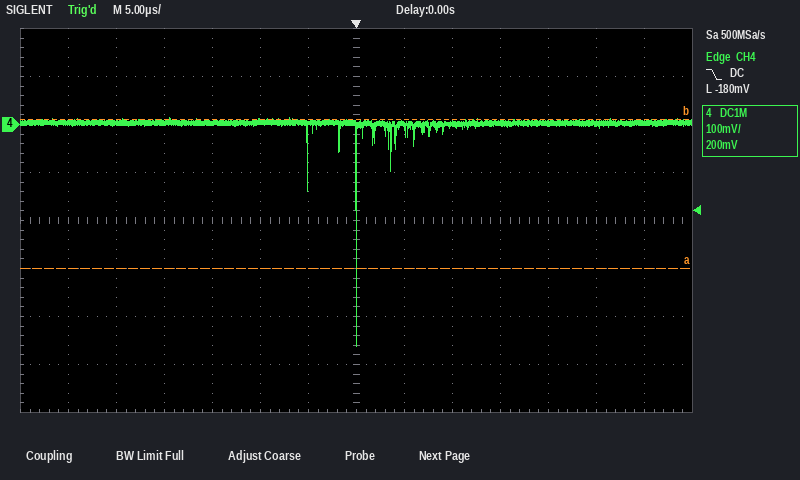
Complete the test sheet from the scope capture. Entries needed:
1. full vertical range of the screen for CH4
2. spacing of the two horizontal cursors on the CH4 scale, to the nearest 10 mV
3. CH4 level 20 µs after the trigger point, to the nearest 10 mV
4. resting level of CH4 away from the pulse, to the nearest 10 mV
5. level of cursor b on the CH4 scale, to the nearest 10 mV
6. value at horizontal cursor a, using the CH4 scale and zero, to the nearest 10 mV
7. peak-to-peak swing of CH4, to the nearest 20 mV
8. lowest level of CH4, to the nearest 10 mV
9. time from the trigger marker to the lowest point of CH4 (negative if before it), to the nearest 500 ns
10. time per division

800 mV
310 mV
0 mV
0 mV
10 mV
-300 mV
480 mV
-460 mV
0.0 µs
5 µs
